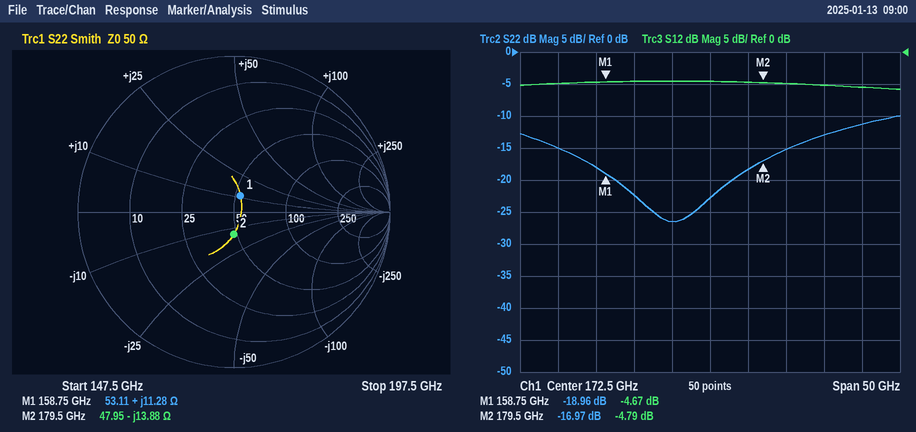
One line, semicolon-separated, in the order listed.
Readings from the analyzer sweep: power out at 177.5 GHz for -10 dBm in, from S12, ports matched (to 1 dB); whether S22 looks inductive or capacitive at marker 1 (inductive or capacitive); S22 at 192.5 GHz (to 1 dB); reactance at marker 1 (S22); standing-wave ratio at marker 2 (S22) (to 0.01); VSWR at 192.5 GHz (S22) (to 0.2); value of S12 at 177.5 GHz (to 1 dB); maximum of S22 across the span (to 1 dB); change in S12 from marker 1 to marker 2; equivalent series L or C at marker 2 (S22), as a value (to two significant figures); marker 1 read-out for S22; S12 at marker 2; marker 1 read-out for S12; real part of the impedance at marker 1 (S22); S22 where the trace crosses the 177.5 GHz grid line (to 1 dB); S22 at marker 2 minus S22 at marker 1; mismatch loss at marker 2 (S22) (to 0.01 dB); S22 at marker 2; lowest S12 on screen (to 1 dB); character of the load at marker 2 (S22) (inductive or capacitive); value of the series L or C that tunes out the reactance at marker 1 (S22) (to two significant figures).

-15 dBm; inductive; -11 dB; +11.28 Ω; 1.33; 1.8; -5 dB; -10 dB; -0.12 dB; 64 fF; -18.96 dB; -4.79 dB; -4.67 dB; 53.11 Ω; -18 dB; 1.99 dB; 0.09 dB; -16.97 dB; -6 dB; capacitive; 89 fF
